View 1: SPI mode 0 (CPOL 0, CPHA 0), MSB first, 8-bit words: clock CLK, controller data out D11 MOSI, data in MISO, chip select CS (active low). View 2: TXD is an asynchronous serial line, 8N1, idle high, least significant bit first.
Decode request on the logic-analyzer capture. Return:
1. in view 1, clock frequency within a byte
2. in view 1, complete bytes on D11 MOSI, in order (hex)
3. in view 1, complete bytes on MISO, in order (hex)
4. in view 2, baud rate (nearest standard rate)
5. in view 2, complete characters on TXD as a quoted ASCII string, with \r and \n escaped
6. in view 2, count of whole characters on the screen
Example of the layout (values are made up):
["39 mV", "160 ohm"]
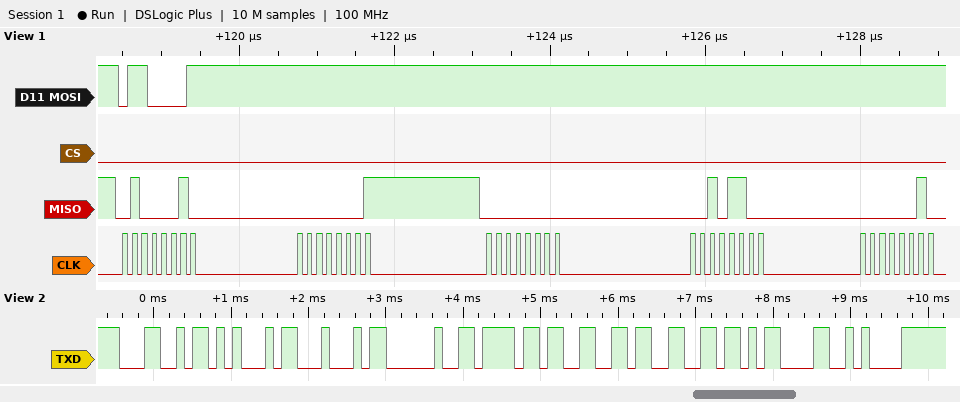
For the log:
["8 MHz", "61 FF FF FF FF", "42 01 00 2C 02", "9600 baud", "\"LED off\\r\\n\"", "9"]
